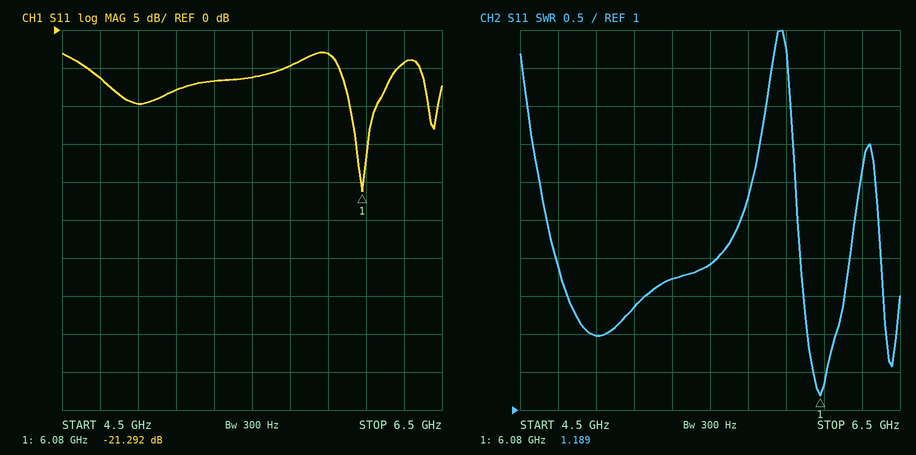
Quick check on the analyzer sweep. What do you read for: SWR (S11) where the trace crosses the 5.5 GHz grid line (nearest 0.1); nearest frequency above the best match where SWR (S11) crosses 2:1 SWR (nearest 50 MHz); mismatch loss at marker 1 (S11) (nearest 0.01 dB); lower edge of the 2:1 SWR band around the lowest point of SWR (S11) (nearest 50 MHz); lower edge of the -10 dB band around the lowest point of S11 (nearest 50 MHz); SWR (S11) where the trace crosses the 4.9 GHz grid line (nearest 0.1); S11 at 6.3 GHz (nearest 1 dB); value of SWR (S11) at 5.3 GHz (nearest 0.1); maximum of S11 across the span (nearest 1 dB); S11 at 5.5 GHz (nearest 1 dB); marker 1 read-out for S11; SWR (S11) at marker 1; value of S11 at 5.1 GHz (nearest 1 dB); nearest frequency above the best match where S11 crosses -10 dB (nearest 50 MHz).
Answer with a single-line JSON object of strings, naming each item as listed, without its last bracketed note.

{"SWR (S11) where the trace crosses the 5.5 GHz grid line": "2.9", "nearest frequency above the best match where SWR (S11) crosses 2:1 SWR": "6.15 GHz", "mismatch loss at marker 1 (S11)": "0.03 dB", "lower edge of the 2:1 SWR band around the lowest point of SWR (S11)": "6.00 GHz", "lower edge of the -10 dB band around the lowest point of S11": "6.00 GHz", "SWR (S11) where the trace crosses the 4.9 GHz grid line": "2.0", "S11 at 6.3 GHz": "-4 dB", "value of SWR (S11) at 5.3 GHz": "2.7", "maximum of S11 across the span": "-3 dB", "S11 at 5.5 GHz": "-6 dB", "marker 1 read-out for S11": "-21.292 dB", "SWR (S11) at marker 1": "1.189", "value of S11 at 5.1 GHz": "-8 dB", "nearest frequency above the best match where S11 crosses -10 dB": "6.15 GHz"}
